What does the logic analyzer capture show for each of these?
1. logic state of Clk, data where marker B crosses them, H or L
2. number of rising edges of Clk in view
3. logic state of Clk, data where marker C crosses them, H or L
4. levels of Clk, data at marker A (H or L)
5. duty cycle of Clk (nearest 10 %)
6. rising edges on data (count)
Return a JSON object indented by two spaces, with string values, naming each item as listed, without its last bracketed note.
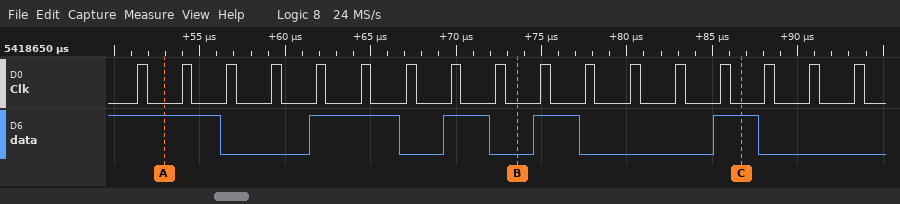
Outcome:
{
  "logic state of Clk, data where marker B crosses them, H or L": "Clk=L, data=L",
  "number of rising edges of Clk in view": "17",
  "logic state of Clk, data where marker C crosses them, H or L": "Clk=L, data=H",
  "levels of Clk, data at marker A": "Clk=L, data=H",
  "duty cycle of Clk": "20 %",
  "rising edges on data": "4"
}
